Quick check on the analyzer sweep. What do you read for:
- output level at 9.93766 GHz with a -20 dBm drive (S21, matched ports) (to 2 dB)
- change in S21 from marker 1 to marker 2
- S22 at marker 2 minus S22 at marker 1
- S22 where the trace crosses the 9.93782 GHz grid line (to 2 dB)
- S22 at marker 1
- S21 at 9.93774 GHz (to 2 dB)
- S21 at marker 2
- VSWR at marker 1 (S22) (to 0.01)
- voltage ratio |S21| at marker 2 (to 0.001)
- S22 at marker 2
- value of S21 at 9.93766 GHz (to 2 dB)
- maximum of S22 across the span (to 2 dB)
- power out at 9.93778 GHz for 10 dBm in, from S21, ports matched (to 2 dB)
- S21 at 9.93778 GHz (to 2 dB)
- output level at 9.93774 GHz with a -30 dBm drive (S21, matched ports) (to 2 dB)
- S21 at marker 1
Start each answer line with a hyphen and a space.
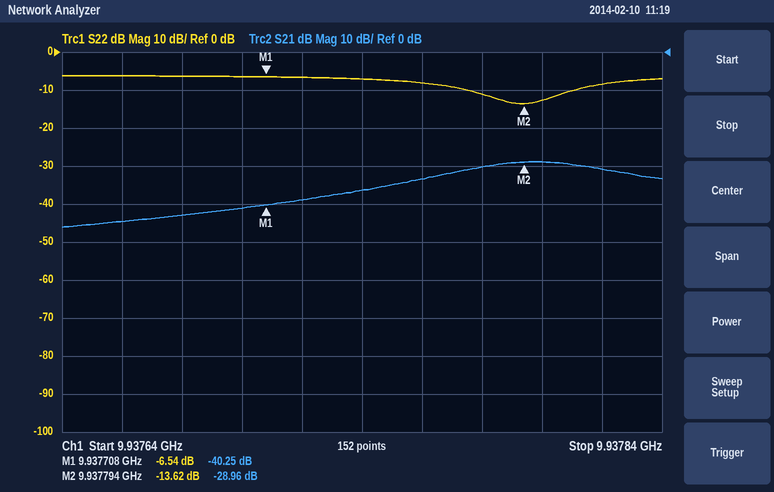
- -64 dBm
- 11.29 dB
- -7.08 dB
- -8 dB
- -6.54 dB
- -36 dB
- -28.96 dB
- 2.78
- 0.036
- -13.62 dB
- -44 dB
- -6 dB
- -20 dBm
- -30 dB
- -66 dBm
- -40.25 dB
